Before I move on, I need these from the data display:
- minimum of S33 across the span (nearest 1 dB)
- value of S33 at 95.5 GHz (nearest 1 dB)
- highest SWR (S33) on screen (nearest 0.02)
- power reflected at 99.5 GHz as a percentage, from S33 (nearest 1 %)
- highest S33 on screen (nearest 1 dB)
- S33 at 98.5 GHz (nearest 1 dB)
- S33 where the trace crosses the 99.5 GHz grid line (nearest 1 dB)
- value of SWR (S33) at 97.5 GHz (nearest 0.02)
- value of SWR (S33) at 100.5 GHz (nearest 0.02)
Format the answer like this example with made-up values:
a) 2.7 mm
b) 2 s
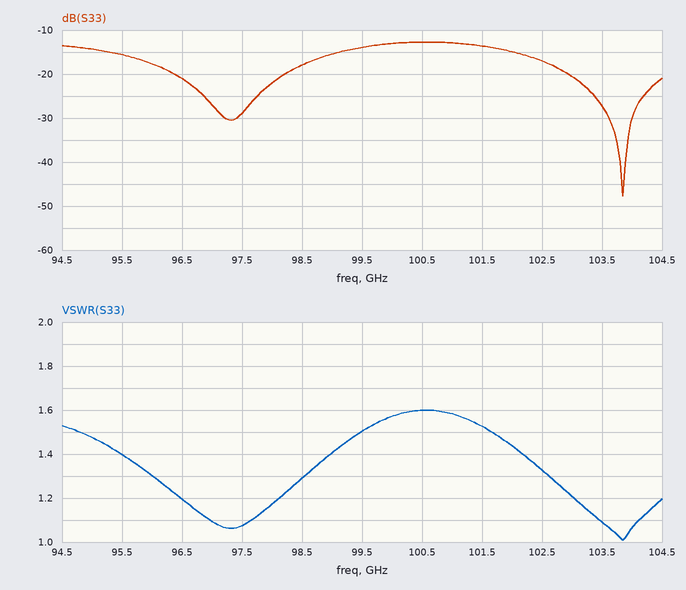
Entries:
a) -48 dB
b) -16 dB
c) 1.60
d) 4 %
e) -13 dB
f) -18 dB
g) -14 dB
h) 1.08
i) 1.60
